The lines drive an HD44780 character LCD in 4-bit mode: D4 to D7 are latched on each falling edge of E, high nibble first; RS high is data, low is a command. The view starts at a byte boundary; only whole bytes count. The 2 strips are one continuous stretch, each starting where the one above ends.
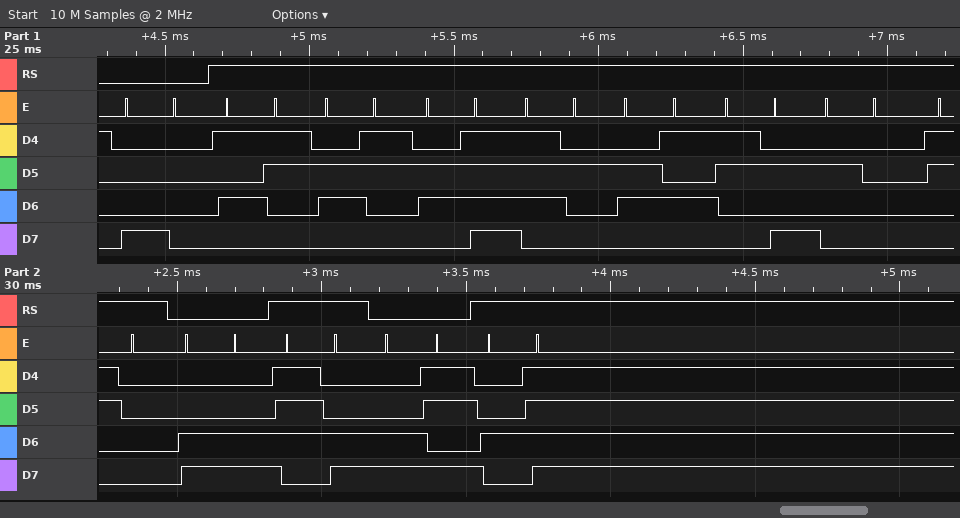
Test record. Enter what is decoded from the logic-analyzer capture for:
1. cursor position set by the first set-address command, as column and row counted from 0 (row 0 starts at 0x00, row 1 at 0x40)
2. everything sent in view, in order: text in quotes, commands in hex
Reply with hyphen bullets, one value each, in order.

- column 0, row 0
- 0x80 "Score: 0" 0xCC "|" 0xCB "O"
